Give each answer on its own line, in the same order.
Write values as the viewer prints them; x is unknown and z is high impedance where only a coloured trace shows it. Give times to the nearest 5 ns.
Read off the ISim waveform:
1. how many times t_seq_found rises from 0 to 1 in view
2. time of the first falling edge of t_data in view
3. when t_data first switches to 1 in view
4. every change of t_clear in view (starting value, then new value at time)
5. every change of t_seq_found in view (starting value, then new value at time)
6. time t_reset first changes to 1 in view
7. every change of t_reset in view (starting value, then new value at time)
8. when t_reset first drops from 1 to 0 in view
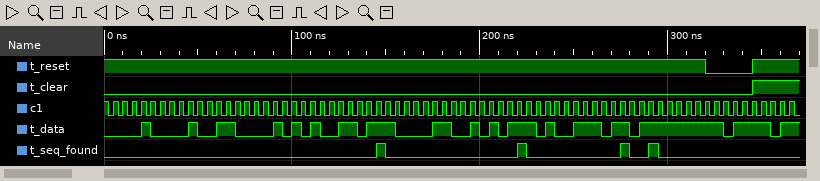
4
25 ns
20 ns
0, 1 at 345 ns
0, 1 at 145 ns, 0 at 150 ns, 1 at 220 ns, 0 at 225 ns, 1 at 275 ns, 0 at 280 ns, 1 at 290 ns, 0 at 295 ns
345 ns
1, 0 at 320 ns, 1 at 345 ns
320 ns
